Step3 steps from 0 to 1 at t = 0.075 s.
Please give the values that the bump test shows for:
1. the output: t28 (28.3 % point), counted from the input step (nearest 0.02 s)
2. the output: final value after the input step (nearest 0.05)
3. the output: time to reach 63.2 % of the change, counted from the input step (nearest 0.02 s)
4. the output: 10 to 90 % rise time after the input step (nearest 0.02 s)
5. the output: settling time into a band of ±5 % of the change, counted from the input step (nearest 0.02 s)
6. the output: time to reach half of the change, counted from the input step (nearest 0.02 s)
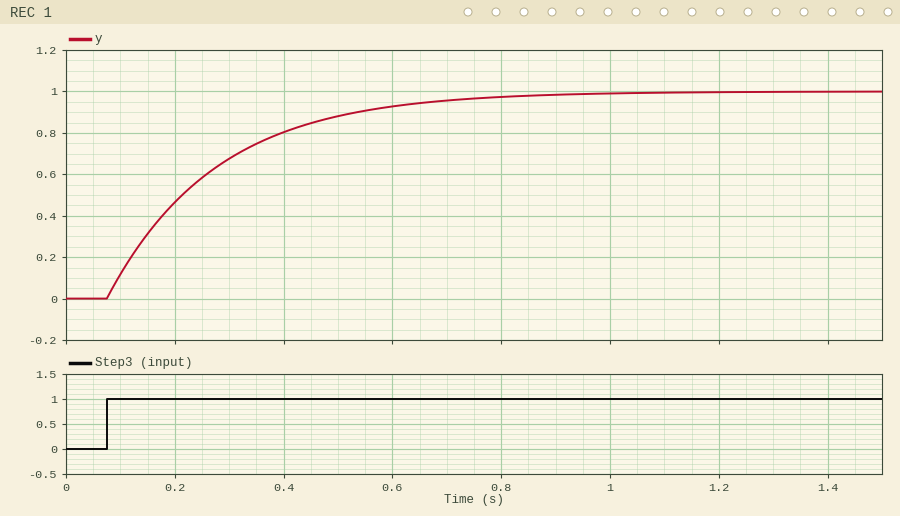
0.06 s
1.00
0.20 s
0.44 s
0.60 s
0.14 s
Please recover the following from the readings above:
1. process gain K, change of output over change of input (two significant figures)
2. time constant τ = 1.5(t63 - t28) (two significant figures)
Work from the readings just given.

1.0
0.21 s
